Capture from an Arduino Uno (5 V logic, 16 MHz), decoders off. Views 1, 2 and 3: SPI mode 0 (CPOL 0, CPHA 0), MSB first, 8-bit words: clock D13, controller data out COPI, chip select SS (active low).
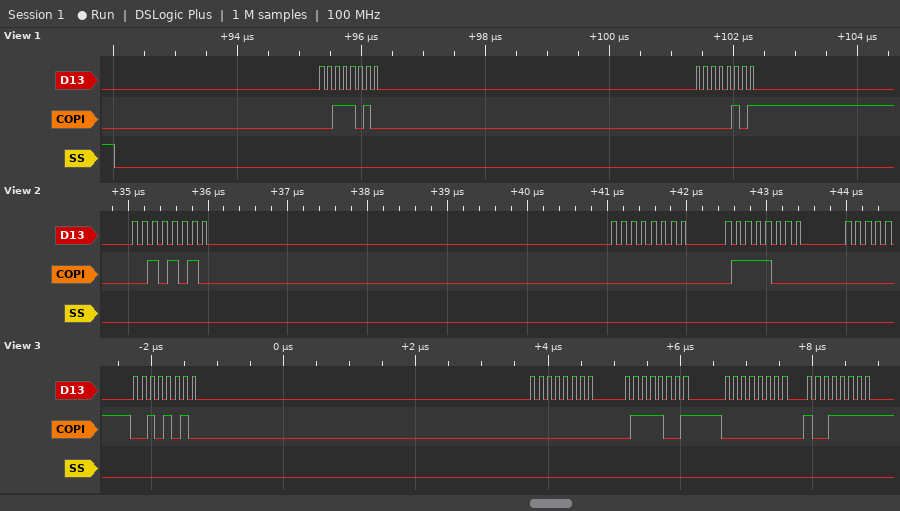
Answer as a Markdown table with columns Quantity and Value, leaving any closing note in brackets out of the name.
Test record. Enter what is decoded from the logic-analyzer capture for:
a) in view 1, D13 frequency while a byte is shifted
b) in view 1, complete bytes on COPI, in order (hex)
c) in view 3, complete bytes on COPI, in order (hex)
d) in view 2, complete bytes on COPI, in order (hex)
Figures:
| Quantity | Value |
|---|---|
| in view 1, D13 frequency while a byte is shifted | 8 MHz |
| in view 1, complete bytes on COPI, in order | 3A 05 |
| in view 3, complete bytes on COPI, in order | 0x2A 0x00 0x79 0x00 0x9F |
| in view 2, complete bytes on COPI, in order | 2A 00 78 |
